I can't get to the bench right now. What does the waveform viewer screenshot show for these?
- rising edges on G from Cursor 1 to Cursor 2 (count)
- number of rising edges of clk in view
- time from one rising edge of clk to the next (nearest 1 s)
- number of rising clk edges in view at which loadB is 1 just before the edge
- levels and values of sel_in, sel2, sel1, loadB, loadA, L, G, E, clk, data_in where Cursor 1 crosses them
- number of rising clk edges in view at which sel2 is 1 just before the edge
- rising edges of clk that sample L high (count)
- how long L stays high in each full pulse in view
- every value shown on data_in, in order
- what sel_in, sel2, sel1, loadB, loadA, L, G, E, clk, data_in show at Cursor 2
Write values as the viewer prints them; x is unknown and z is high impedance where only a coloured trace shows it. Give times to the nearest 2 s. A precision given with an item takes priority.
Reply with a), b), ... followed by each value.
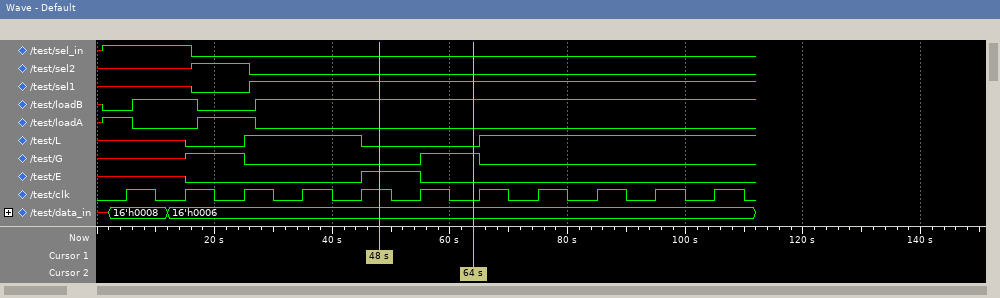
a) 1
b) 11
c) 10 s
d) 9
e) sel_in=0, sel2=0, sel1=1, loadB=1, loadA=0, L=0, G=0, E=1, clk=1, data_in=16'h0006
f) 1
g) 6
h) 20 s
i) x, 16'h0008, 16'h0006
j) sel_in=0, sel2=0, sel1=1, loadB=1, loadA=0, L=0, G=1, E=0, clk=0, data_in=16'h0006
